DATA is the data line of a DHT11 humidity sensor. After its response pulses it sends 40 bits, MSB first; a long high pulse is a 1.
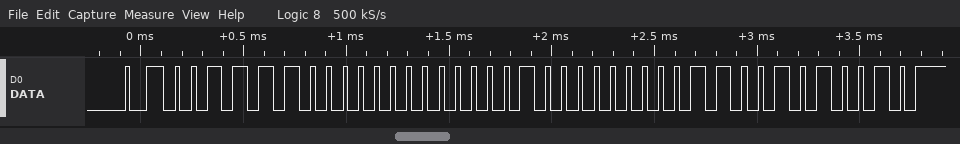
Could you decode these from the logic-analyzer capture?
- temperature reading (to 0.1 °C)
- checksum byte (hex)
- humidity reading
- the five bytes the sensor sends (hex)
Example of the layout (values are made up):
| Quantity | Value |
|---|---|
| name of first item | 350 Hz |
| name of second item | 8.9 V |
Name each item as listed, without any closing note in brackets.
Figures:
| Quantity | Value |
|---|---|
| temperature reading | 16.6 °C |
| checksum byte | 0x52 |
| humidity reading | 60 % |
| the five bytes the sensor sends | 3C 00 10 06 52 |
